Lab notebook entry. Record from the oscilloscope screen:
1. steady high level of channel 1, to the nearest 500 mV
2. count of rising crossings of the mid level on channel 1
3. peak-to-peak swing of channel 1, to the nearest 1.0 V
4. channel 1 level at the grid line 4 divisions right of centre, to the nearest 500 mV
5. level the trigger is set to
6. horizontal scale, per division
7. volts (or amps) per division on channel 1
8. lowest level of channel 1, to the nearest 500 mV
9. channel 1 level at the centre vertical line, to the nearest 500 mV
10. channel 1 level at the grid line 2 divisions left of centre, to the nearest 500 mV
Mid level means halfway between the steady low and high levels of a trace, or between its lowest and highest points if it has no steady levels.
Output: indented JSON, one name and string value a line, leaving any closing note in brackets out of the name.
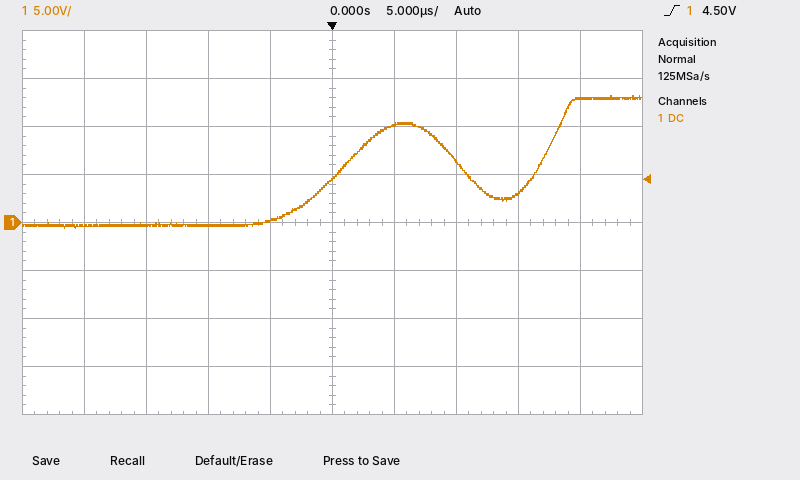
{
  "steady high level of channel 1, to the nearest 500 mV": "13.0 V",
  "count of rising crossings of the mid level on channel 1": "2",
  "peak-to-peak swing of channel 1, to the nearest 1.0 V": "14.0 V",
  "channel 1 level at the grid line 4 divisions right of centre, to the nearest 500 mV": "13.0 V",
  "level the trigger is set to": "4.50 V",
  "horizontal scale, per division": "5 µs",
  "volts (or amps) per division on channel 1": "5 V",
  "lowest level of channel 1, to the nearest 500 mV": "-500 mV",
  "channel 1 level at the centre vertical line, to the nearest 500 mV": "4.5 V",
  "channel 1 level at the grid line 2 divisions left of centre, to the nearest 500 mV": "-500 mV"
}
